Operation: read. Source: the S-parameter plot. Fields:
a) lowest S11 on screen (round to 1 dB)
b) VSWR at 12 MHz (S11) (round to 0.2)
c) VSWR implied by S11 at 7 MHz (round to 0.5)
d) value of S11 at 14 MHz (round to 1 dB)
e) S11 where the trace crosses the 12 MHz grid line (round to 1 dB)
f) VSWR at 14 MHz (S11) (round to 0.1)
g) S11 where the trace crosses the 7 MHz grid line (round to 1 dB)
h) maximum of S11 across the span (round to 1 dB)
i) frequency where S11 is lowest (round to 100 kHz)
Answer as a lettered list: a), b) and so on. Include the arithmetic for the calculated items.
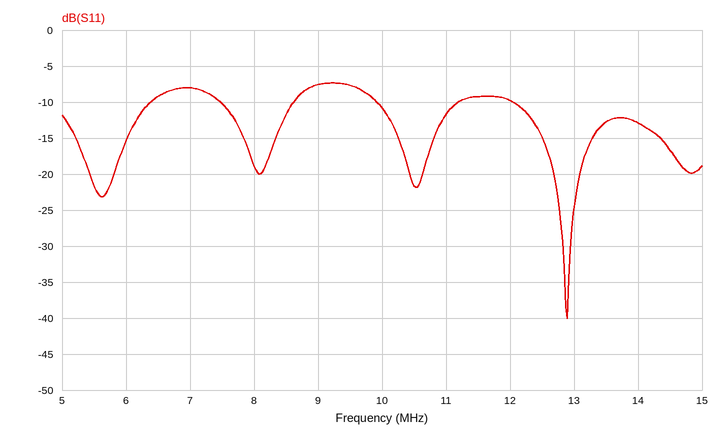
a) -40 dB
b) |Γ| = 10^(-10/20) = 0.3162; VSWR = (1 + 0.3162)/(1 − 0.3162) ≈ 1.92, so 2.0 to the nearest 0.2
c) |Γ| = 10^(-8/20) = 0.3981; VSWR = (1 + 0.3981)/(1 − 0.3981) ≈ 2.32, so 2.5 to the nearest 0.5
d) -13 dB
e) -10 dB
f) |Γ| = 10^(-13/20) = 0.2239; VSWR = (1 + 0.2239)/(1 − 0.2239) ≈ 1.6
g) -8 dB
h) -7 dB
i) 12.9 MHz
